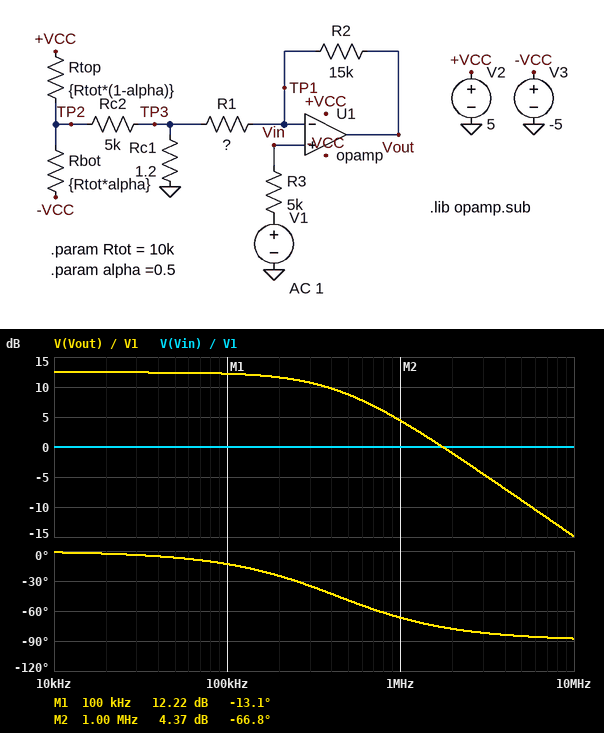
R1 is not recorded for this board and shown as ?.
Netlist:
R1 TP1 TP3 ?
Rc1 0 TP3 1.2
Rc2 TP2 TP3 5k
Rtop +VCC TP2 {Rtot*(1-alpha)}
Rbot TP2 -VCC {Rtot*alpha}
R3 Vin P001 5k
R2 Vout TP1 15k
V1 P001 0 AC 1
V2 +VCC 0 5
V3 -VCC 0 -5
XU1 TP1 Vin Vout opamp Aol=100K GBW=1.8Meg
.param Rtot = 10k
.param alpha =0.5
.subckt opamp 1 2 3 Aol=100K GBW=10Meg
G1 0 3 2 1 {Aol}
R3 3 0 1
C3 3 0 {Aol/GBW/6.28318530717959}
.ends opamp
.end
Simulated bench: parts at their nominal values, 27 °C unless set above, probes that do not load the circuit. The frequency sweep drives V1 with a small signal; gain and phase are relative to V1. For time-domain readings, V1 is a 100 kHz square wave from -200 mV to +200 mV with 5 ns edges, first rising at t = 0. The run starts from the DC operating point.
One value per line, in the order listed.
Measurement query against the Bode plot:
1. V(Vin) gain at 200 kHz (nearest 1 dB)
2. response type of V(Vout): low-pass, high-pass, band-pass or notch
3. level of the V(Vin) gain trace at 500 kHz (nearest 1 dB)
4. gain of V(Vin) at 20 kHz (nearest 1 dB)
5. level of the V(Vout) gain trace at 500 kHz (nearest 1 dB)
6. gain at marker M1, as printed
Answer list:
0 dB
low-pass
0 dB
0 dB
9 dB
12.22 dB
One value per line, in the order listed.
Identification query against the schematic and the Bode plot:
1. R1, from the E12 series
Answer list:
4.7 kΩ
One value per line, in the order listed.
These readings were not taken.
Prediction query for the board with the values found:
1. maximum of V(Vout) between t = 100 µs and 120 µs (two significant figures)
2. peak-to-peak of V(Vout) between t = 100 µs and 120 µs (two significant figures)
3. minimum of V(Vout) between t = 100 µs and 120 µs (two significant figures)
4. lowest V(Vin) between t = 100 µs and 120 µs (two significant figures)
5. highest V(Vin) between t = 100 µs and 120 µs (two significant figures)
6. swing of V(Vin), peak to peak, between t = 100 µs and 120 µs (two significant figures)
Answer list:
840 mV
1.7 V
-840 mV
-200 mV
200 mV
400 mV
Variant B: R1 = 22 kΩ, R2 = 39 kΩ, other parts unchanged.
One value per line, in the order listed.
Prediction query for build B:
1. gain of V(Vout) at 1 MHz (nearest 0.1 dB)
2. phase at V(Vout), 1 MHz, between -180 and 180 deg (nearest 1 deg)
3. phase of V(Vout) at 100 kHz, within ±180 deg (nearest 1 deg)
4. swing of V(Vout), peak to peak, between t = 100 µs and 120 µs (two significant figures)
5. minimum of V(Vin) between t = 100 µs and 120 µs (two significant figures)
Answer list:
3.6 dB
-57 deg
-9 deg
1.1 V
-200 mV
